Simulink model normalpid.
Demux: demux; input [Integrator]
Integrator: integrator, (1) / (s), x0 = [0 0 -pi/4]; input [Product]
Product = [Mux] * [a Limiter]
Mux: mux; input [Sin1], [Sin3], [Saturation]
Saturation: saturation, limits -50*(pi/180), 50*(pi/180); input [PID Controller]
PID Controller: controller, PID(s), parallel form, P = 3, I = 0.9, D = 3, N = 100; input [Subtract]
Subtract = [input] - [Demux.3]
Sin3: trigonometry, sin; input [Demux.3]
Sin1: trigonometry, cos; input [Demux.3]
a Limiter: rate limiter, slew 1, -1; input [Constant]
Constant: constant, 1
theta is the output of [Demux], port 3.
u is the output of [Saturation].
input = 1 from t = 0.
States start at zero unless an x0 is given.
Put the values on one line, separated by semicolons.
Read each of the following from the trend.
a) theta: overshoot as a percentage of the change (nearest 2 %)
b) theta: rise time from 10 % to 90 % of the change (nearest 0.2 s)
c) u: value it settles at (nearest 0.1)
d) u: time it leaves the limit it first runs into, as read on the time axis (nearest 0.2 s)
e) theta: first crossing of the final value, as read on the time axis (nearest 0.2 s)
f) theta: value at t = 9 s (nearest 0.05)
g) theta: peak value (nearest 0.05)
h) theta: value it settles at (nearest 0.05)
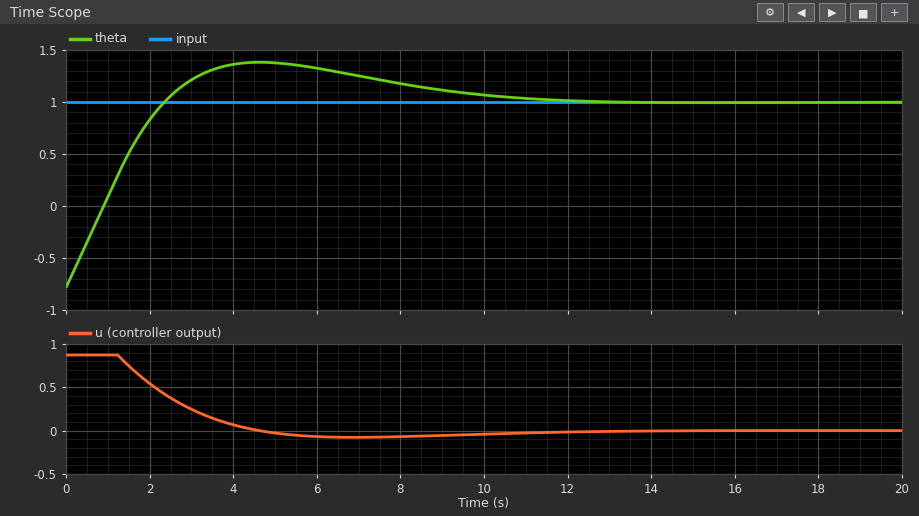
22 %; 1.8 s; 0.0; 1.2 s; 2.4 s; 1.10; 1.40; 1.00
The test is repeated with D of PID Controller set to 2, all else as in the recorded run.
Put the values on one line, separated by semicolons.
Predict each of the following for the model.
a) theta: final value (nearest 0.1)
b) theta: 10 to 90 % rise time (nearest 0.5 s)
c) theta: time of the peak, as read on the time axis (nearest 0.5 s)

1.0; 1.5 s; 4.0 s
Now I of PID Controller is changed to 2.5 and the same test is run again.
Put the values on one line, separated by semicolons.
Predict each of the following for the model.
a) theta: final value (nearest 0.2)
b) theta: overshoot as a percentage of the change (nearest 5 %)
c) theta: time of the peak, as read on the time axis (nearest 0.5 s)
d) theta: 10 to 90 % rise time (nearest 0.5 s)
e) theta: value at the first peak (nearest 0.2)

1.0; 45 %; 3.5 s; 1.5 s; 1.8
